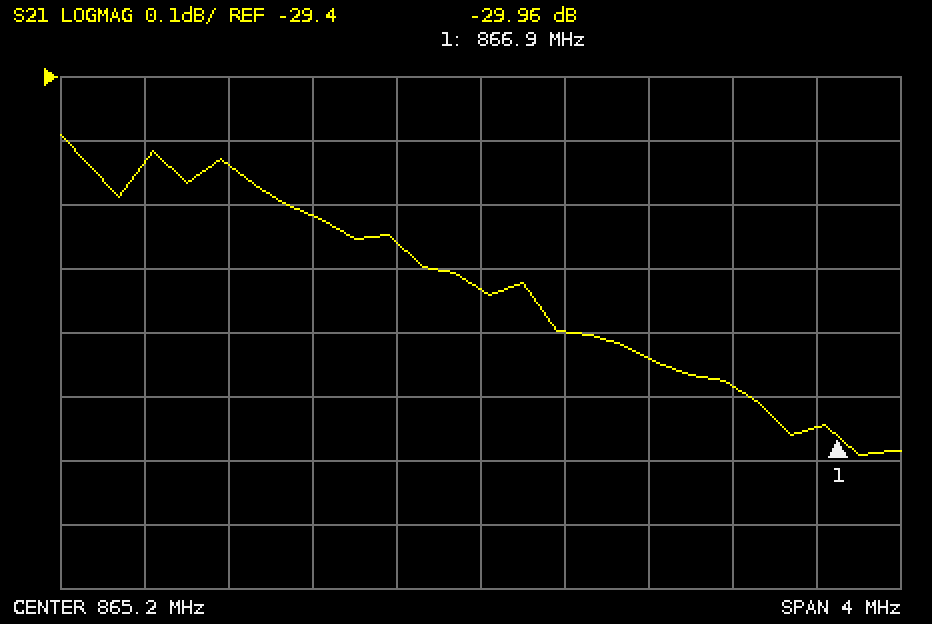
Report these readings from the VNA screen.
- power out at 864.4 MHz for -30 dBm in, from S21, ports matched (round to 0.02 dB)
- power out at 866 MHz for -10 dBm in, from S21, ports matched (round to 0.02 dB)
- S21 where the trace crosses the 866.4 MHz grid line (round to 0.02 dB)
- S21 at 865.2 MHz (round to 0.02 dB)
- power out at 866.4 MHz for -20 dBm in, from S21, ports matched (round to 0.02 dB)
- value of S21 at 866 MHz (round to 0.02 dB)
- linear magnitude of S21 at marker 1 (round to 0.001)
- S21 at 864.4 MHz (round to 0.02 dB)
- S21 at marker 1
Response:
-59.62 dBm
-39.84 dBm
-29.88 dB
-29.74 dB
-49.88 dBm
-29.84 dB
0.032
-29.62 dB
-29.96 dB
